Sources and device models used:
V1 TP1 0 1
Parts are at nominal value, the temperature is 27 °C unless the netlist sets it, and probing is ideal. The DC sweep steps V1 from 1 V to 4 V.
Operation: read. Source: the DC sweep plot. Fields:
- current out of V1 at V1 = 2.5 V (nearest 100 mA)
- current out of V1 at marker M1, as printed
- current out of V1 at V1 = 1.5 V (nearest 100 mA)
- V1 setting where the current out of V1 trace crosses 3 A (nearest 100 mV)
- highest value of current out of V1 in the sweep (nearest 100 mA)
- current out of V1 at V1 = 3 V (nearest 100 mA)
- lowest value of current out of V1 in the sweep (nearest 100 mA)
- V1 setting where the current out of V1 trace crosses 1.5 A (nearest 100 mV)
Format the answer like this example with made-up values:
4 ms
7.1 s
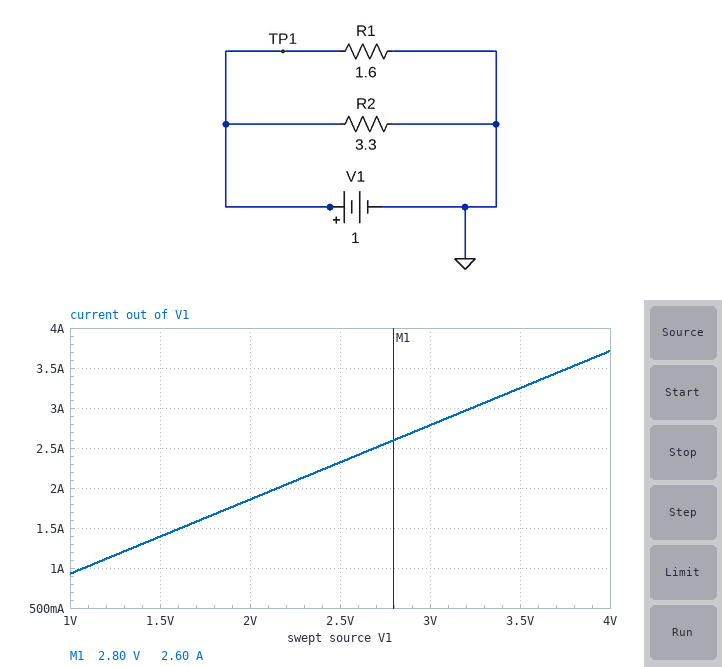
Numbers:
2.3 A
2.60 A
1.4 A
3.2 V
3.7 A
2.8 A
900 mA
1.6 V
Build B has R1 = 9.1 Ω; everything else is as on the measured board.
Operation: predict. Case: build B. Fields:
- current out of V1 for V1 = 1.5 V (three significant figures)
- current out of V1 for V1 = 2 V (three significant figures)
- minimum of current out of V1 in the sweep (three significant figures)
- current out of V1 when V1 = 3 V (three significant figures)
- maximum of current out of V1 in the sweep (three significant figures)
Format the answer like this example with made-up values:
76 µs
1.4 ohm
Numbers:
619 mA
826 mA
413 mA
1.24 A
1.65 A
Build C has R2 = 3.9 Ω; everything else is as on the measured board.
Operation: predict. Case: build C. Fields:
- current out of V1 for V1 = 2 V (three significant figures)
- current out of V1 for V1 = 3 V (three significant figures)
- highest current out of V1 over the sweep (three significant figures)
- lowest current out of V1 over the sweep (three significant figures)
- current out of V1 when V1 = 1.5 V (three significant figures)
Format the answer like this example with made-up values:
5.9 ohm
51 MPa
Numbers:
1.76 A
2.64 A
3.53 A
881 mA
1.32 A
